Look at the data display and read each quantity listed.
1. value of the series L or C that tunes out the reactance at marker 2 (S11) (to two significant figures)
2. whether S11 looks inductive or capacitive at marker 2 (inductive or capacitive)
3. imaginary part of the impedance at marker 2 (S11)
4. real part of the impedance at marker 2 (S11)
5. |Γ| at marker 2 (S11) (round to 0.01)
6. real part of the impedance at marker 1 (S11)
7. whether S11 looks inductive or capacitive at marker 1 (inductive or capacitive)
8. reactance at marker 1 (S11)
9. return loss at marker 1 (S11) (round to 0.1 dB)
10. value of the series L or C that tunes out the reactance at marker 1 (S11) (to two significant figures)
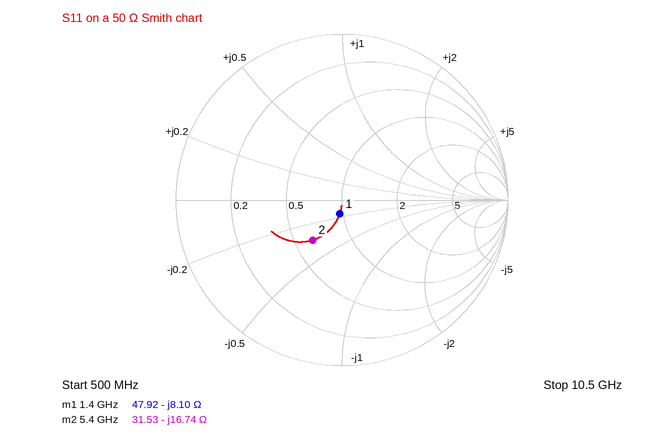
490 pH
capacitive
-16.74 Ω
31.53 Ω
0.30
47.92 Ω
capacitive
-8.10 Ω
21.4 dB
920 pH
